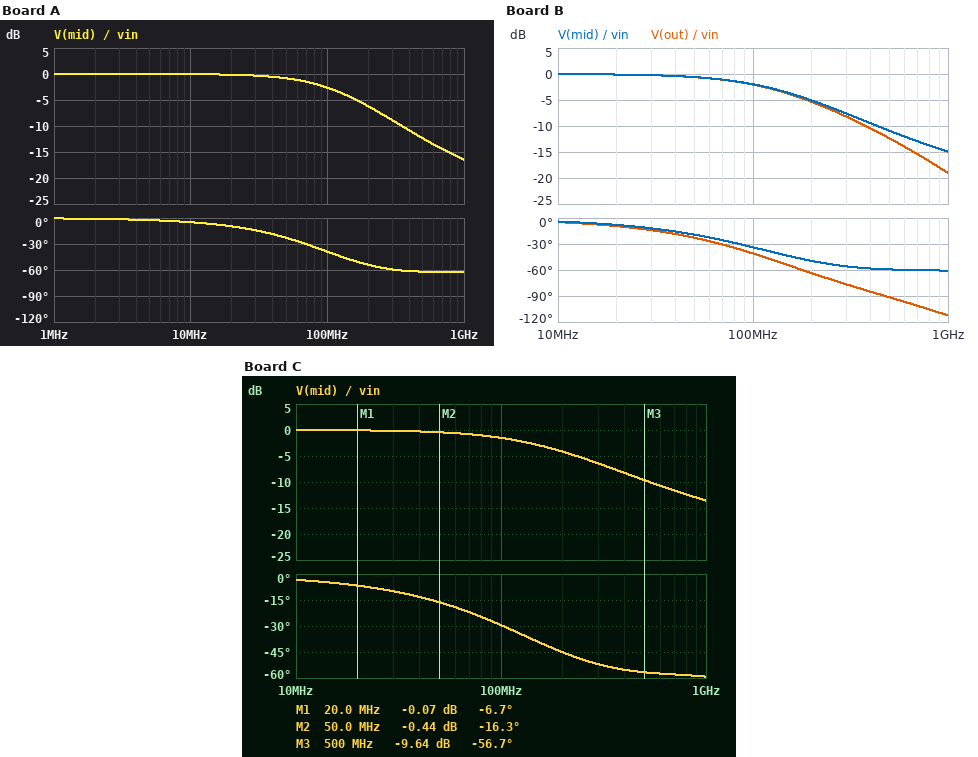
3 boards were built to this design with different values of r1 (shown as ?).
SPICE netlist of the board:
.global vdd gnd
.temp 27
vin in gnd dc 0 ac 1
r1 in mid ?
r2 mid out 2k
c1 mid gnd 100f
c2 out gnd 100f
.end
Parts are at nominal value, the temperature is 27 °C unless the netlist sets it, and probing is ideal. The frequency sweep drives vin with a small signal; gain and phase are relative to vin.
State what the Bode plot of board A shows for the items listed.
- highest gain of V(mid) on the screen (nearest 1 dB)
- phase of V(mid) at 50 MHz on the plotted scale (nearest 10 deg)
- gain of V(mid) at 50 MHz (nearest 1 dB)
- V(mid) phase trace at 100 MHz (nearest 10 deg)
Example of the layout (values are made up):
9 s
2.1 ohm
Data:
0 dB
-20 deg
-1 dB
-40 deg
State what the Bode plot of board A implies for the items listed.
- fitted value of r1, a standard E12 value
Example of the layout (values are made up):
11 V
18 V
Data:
6.8 kΩ
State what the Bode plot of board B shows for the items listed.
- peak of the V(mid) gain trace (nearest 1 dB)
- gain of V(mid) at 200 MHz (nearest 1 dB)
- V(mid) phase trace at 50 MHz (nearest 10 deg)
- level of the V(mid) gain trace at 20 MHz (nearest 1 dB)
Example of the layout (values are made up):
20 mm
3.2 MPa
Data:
0 dB
-5 dB
-20 deg
0 dB
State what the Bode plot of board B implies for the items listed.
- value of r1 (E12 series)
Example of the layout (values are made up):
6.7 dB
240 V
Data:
5.6 kΩ
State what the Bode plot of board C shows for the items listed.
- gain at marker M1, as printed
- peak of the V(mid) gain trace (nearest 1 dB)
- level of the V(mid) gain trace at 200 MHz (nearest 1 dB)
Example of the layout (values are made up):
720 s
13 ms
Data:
-0.07 dB
0 dB
-4 dB
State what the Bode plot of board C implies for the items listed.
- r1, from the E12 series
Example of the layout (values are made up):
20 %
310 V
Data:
4.7 kΩ
